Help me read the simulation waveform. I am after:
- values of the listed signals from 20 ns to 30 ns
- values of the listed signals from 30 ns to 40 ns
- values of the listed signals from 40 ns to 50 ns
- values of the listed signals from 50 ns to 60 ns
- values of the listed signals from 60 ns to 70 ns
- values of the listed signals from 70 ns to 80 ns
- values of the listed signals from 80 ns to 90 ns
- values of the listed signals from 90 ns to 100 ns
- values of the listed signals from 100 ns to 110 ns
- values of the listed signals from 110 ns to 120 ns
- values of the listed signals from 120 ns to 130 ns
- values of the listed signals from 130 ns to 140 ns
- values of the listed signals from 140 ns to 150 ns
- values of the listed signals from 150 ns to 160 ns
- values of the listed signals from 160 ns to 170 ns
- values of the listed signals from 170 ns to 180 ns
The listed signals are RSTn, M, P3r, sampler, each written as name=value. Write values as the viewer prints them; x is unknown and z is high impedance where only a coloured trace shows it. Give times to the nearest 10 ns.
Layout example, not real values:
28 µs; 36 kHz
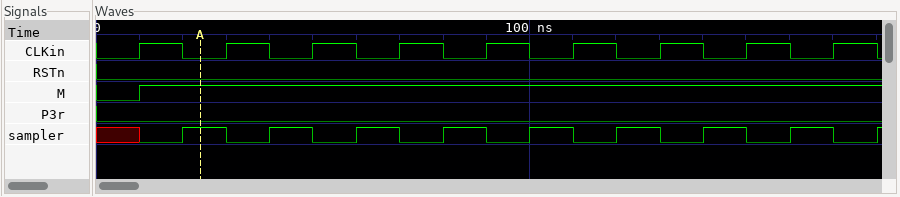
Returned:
RSTn=0, M=1, P3r=0, sampler=1; RSTn=0, M=1, P3r=0, sampler=0; RSTn=0, M=1, P3r=0, sampler=1; RSTn=0, M=1, P3r=0, sampler=0; RSTn=0, M=1, P3r=0, sampler=1; RSTn=0, M=1, P3r=0, sampler=0; RSTn=0, M=1, P3r=0, sampler=1; RSTn=0, M=1, P3r=0, sampler=0; RSTn=0, M=1, P3r=0, sampler=1; RSTn=0, M=1, P3r=0, sampler=0; RSTn=0, M=1, P3r=0, sampler=1; RSTn=0, M=1, P3r=0, sampler=0; RSTn=0, M=1, P3r=0, sampler=1; RSTn=0, M=1, P3r=0, sampler=0; RSTn=0, M=1, P3r=0, sampler=1; RSTn=0, M=1, P3r=0, sampler=0
